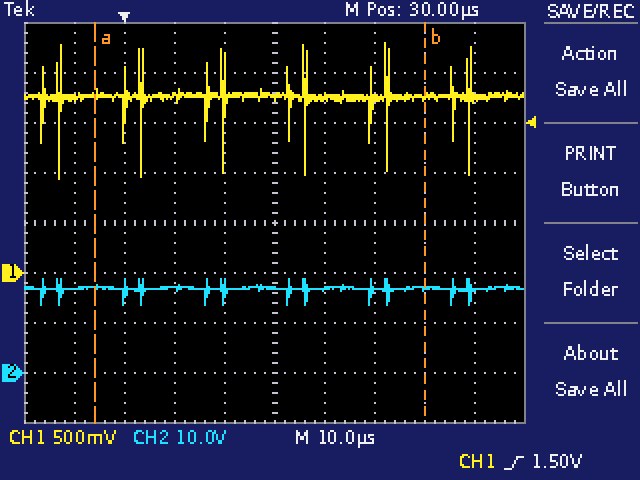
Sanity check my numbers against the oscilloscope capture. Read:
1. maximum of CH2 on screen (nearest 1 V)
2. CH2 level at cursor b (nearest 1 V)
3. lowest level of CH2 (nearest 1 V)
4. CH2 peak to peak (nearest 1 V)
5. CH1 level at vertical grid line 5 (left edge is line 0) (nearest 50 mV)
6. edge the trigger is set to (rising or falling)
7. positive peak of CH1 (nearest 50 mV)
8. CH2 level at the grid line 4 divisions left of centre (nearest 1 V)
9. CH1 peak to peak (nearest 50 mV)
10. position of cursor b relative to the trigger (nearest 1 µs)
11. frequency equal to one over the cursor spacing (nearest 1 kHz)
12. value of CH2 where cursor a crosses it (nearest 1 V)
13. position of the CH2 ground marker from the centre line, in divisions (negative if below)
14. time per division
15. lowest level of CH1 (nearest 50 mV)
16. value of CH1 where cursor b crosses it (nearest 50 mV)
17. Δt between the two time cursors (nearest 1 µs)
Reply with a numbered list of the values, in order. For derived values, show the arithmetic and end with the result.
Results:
1. 19 V
2. 17 V
3. 14 V
4. 19 V − (14 V) = 5 V
5. 1.75 V
6. rising
7. 2.30 V
8. 17 V
9. 2.30 V − (950 mV) = 1.35 V
10. +60 µs
11. 1 / 66 µs ≈ 15 kHz
12. 17 V
13. -3.0 div
14. 10 µs
15. 950 mV
16. 1.75 V
17. 66 µs
